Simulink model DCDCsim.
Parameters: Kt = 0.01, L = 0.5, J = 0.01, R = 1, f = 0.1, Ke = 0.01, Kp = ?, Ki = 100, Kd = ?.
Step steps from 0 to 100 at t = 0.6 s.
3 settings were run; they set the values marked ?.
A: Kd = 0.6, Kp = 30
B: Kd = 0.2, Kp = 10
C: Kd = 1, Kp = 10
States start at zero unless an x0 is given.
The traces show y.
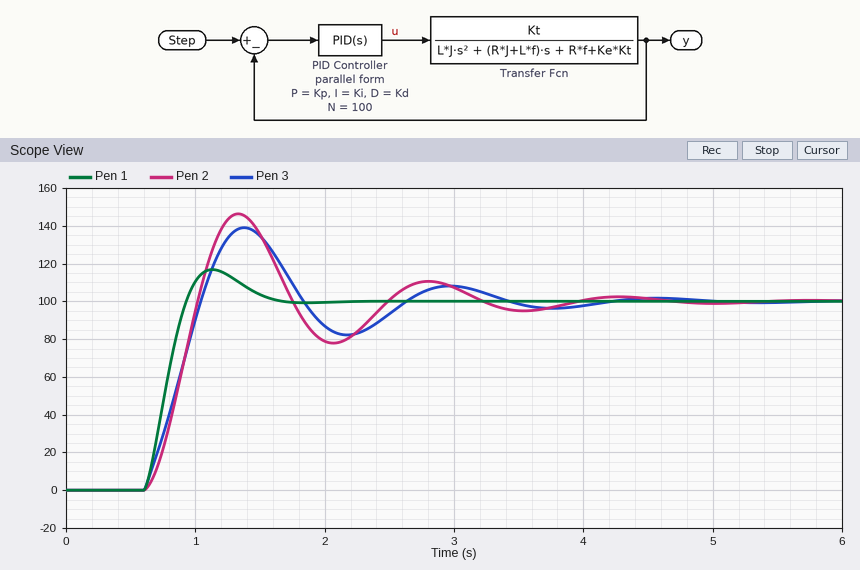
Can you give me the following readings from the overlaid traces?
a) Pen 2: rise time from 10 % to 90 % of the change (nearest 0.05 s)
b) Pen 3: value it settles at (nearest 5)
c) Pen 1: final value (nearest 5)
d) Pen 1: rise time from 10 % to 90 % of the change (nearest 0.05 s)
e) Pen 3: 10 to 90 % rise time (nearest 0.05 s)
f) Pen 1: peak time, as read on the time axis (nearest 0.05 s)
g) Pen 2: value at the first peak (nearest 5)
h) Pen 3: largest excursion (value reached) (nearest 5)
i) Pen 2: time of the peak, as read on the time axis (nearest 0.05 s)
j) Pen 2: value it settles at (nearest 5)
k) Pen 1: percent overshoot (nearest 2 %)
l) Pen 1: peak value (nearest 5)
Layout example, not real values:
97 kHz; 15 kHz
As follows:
0.30 s; 100; 100; 0.25 s; 0.35 s; 1.15 s; 145; 140; 1.35 s; 100; 16 %; 115
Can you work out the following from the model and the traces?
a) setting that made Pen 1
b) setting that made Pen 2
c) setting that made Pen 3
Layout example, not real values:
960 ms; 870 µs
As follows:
A; B; C
